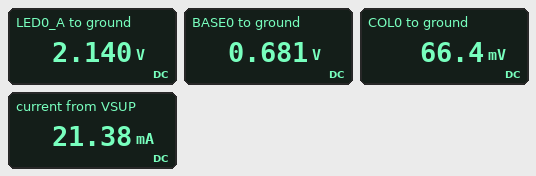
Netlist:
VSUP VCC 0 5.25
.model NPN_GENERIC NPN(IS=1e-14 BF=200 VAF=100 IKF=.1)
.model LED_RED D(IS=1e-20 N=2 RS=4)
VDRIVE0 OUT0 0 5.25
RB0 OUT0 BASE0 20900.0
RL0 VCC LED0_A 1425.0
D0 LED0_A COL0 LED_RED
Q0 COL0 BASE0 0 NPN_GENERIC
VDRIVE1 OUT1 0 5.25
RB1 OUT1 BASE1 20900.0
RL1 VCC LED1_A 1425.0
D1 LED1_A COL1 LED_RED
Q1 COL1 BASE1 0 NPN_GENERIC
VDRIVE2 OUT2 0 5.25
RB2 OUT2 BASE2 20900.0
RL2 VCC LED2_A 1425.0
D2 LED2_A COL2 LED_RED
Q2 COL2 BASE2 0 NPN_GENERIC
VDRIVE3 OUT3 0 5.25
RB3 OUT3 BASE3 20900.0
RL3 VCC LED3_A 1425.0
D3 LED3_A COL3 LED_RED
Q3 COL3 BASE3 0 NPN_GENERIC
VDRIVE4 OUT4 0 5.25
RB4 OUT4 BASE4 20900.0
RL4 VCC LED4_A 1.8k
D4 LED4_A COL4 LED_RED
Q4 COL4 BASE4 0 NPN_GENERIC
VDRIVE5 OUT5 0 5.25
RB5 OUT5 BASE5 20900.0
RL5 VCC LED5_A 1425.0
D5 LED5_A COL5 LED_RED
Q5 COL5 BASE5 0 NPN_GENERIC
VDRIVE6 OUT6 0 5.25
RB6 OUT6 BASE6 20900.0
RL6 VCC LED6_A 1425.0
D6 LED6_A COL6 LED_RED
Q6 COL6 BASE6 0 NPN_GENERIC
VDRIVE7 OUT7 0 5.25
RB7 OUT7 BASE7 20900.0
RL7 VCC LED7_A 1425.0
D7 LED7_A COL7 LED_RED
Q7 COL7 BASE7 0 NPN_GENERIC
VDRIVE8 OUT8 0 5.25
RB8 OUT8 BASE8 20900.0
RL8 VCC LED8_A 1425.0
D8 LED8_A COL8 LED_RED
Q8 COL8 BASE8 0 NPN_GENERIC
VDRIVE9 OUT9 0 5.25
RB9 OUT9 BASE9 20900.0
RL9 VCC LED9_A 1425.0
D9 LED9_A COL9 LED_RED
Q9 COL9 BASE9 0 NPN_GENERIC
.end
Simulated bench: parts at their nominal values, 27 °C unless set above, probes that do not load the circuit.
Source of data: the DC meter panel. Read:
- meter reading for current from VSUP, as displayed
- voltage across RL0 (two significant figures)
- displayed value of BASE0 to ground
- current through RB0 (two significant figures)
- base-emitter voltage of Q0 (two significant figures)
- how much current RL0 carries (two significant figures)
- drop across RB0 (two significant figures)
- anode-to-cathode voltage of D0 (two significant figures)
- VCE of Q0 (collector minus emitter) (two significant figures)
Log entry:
21.38 mA
3.1 V
0.681 V
220 µA
680 mV
2.2 mA
4.6 V
2.1 V
66 mV
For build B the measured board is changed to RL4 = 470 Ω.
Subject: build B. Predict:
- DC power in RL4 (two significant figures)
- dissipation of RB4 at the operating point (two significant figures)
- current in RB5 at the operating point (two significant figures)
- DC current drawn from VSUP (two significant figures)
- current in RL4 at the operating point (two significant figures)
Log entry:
19 mW
990 µW
220 µA
26 mA
6.4 mA
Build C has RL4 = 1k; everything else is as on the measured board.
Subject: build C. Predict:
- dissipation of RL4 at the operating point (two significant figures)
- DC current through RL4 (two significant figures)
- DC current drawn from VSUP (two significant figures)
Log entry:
9.5 mW
3.1 mA
23 mA
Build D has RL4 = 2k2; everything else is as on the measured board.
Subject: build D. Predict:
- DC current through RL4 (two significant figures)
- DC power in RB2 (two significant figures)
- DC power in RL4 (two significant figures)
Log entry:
1.4 mA
1.0 mW
4.5 mW
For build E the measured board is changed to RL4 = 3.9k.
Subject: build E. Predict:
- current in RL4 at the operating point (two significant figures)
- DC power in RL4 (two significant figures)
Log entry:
820 µA
2.6 mW
